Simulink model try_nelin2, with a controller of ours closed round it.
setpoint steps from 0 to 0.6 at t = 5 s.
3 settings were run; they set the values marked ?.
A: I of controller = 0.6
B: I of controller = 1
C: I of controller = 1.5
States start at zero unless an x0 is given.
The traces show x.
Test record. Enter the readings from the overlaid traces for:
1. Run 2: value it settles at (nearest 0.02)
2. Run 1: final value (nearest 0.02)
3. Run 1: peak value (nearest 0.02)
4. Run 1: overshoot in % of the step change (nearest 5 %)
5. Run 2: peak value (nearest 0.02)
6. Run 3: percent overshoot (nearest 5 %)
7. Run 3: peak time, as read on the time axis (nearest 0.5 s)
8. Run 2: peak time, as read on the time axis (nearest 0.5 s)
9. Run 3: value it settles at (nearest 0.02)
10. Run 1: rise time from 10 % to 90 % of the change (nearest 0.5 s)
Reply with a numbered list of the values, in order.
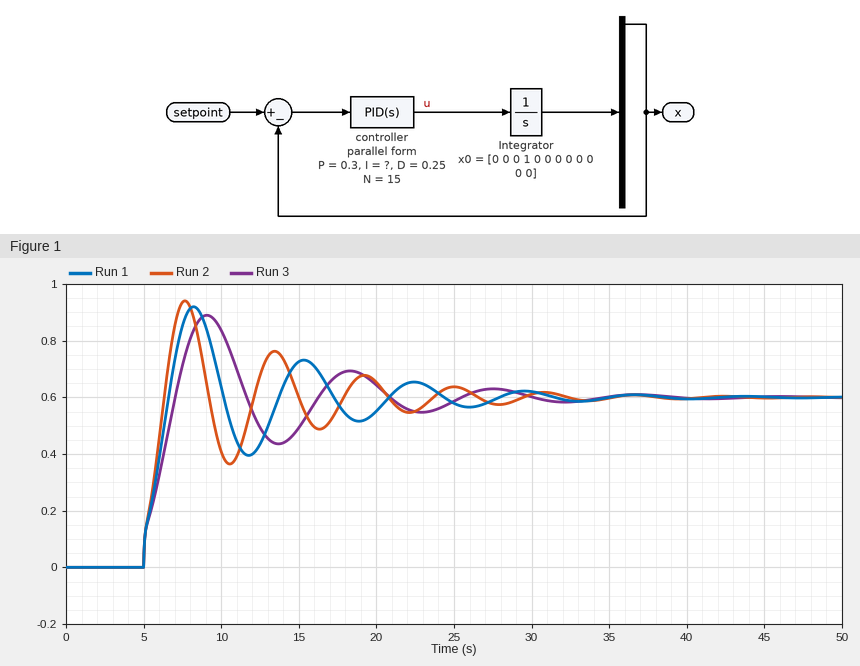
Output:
1. 0.60
2. 0.60
3. 0.92
4. 55 %
5. 0.94
6. 50 %
7. 9.0 s
8. 7.5 s
9. 0.60
10. 1.5 s
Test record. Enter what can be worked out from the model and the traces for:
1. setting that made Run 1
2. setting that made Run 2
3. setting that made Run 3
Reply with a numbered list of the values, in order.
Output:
1. B
2. C
3. A
